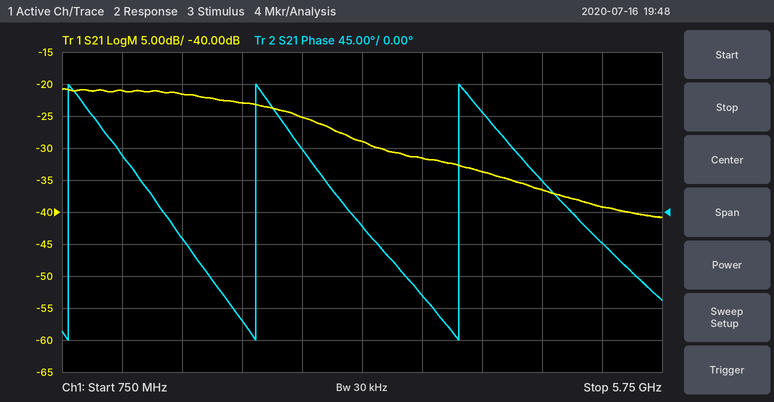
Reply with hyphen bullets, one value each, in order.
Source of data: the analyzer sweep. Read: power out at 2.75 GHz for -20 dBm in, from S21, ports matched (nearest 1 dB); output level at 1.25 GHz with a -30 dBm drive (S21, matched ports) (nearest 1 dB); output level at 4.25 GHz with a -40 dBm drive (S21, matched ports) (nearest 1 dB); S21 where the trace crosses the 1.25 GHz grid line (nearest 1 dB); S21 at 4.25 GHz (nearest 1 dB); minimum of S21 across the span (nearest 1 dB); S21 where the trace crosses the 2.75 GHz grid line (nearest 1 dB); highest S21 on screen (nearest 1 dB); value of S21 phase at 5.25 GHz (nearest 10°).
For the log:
- -45 dBm
- -51 dBm
- -74 dBm
- -21 dB
- -34 dB
- -41 dB
- -25 dB
- -21 dB
- -40°
